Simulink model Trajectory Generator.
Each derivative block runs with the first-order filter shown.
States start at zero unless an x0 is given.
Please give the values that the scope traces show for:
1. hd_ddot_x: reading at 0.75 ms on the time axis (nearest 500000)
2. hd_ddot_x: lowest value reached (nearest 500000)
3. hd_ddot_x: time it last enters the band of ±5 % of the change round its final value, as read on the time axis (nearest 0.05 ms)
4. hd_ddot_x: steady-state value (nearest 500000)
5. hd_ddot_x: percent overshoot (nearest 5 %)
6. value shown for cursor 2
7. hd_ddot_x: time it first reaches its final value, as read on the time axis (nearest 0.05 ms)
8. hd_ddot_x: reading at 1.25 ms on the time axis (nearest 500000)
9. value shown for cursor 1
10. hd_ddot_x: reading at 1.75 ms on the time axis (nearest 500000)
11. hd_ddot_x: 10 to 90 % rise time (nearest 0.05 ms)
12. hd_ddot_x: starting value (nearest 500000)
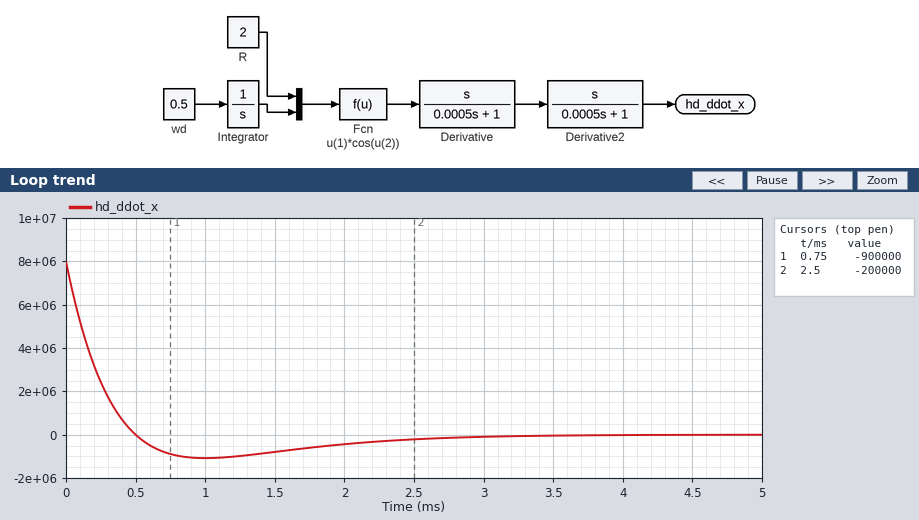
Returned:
-1000000
-1000000
2.05 ms
0
15 %
-200000
0.50 ms
-1000000
-900000
-500000
0.35 ms
8000000
